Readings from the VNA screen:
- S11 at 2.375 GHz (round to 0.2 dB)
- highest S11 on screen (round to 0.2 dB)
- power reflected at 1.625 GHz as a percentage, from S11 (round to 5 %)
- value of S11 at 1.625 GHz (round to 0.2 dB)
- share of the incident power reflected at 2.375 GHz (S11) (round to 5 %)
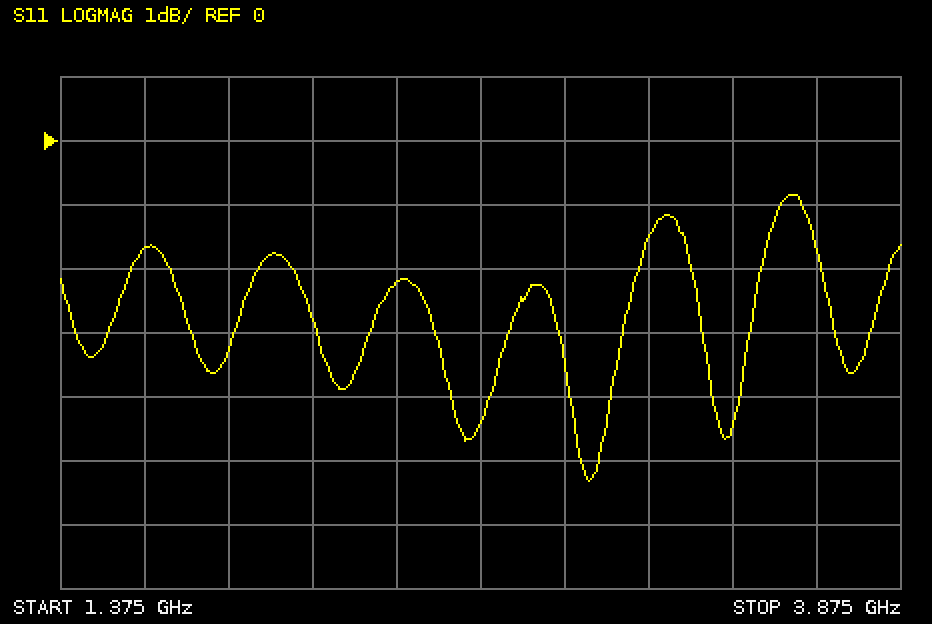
-2.2 dB
-0.8 dB
70 %
-1.6 dB
60 %
